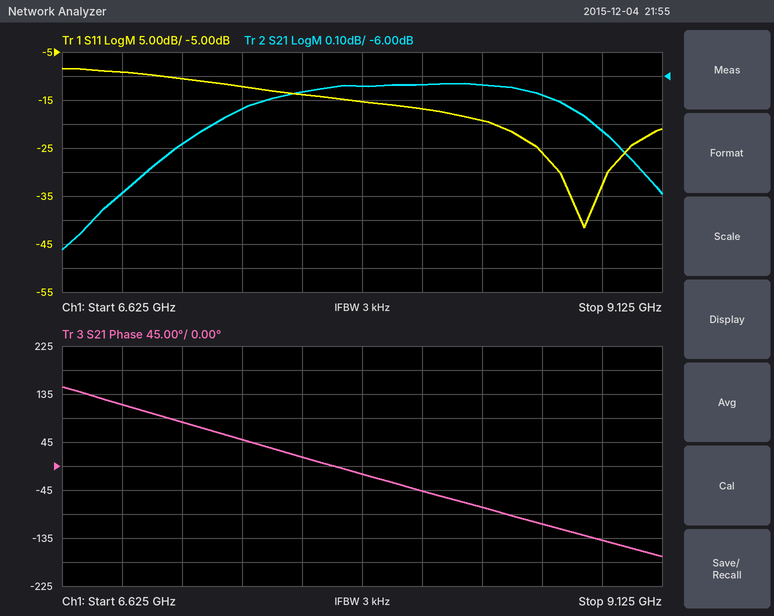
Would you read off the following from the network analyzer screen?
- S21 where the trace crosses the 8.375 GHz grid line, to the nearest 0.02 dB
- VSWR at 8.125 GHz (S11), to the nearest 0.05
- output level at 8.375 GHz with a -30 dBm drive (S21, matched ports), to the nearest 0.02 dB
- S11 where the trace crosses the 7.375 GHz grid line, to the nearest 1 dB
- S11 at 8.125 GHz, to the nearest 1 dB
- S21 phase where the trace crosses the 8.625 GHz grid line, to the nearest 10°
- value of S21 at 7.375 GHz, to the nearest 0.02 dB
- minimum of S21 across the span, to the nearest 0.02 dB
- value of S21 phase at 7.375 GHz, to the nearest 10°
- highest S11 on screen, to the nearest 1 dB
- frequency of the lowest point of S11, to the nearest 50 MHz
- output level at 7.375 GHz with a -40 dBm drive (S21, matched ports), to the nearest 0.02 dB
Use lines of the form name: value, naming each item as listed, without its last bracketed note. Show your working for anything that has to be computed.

S21 where the trace crosses the 8.375 GHz grid line, to the nearest 0.02 dB: -6.04 dB
VSWR at 8.125 GHz (S11), to the nearest 0.05: |Γ| = 10^(-17/20) = 0.1413; VSWR = (1 + 0.1413)/(1 − 0.1413) ≈ 1.33, so 1.35 to the nearest 0.05
output level at 8.375 GHz with a -30 dBm drive (S21, matched ports), to the nearest 0.02 dB: -30 dBm + (-6.04 dB) = -36.04 dBm
S11 where the trace crosses the 7.375 GHz grid line, to the nearest 1 dB: -12 dB
S11 at 8.125 GHz, to the nearest 1 dB: -17 dB
S21 phase where the trace crosses the 8.625 GHz grid line, to the nearest 10°: -110°
value of S21 at 7.375 GHz, to the nearest 0.02 dB: -6.14 dB
minimum of S21 across the span, to the nearest 0.02 dB: -6.72 dB
value of S21 phase at 7.375 GHz, to the nearest 10°: 50°
highest S11 on screen, to the nearest 1 dB: -8 dB
frequency of the lowest point of S11, to the nearest 50 MHz: 8.80 GHz
output level at 7.375 GHz with a -40 dBm drive (S21, matched ports), to the nearest 0.02 dB: -40 dBm + (-6.14 dB) = -46.14 dBm
